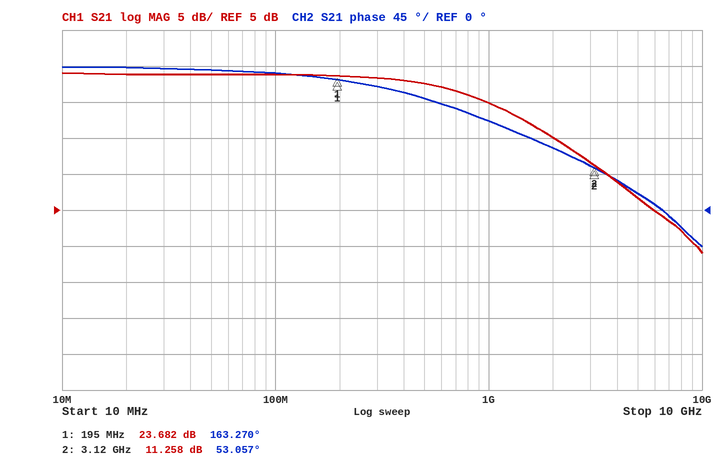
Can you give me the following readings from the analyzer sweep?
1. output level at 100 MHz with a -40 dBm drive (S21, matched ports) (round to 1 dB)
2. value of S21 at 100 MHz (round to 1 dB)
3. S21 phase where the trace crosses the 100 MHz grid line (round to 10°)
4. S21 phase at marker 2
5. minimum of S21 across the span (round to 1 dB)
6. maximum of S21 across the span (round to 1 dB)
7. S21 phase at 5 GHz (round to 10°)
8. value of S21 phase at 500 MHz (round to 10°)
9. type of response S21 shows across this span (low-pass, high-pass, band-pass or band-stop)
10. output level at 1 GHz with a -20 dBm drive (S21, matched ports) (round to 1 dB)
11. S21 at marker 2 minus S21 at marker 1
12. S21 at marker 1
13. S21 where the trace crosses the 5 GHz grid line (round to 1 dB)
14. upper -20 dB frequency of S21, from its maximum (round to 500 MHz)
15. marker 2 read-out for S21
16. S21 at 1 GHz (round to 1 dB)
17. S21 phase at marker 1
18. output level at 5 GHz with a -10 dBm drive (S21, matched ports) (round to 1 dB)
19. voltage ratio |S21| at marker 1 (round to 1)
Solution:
-16 dBm
24 dB
170°
53.057°
-1 dB
24 dB
20°
140°
low-pass
0 dBm
-12.424 dB
23.682 dB
7 dB
6.5 GHz
11.258 dB
20 dB
163.270°
-3 dBm
15
